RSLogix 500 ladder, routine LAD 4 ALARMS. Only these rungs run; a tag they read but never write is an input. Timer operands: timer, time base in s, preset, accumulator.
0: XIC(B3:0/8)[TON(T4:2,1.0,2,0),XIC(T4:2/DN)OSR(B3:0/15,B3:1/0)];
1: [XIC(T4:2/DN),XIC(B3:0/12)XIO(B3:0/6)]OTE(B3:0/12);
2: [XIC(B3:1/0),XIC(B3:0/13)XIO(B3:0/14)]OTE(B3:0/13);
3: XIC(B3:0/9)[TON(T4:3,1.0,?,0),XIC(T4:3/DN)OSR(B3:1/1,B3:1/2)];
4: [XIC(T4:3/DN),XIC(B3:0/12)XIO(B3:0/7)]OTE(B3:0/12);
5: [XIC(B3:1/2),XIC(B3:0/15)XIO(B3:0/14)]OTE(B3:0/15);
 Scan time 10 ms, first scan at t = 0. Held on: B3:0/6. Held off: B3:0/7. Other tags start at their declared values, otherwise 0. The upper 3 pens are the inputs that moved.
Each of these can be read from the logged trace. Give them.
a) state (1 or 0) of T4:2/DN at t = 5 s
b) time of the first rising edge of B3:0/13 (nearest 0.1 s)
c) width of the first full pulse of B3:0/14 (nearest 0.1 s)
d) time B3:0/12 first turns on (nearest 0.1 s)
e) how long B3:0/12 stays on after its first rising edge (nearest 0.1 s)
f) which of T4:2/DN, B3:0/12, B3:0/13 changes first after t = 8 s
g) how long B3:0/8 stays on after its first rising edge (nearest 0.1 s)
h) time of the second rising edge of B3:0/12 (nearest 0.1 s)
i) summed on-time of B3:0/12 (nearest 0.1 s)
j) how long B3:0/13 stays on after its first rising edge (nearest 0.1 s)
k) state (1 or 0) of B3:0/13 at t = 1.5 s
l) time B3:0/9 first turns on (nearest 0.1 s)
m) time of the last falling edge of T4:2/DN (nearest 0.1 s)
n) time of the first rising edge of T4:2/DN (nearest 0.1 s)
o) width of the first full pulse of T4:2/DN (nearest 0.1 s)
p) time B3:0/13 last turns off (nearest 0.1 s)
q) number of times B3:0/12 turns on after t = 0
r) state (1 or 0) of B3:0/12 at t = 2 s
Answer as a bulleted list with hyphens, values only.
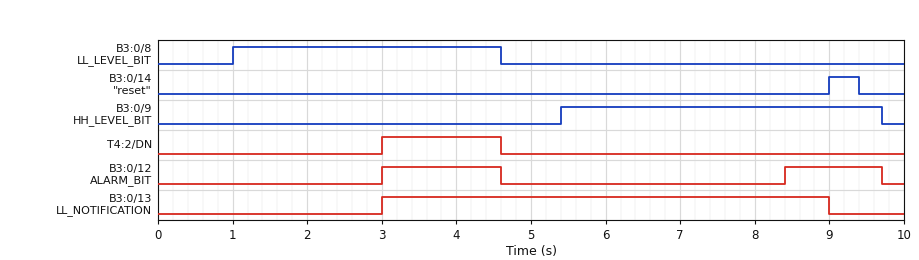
- 0
- 3.0 s
- 0.4 s
- 3.0 s
- 1.6 s
- B3:0/12
- 3.6 s
- 8.4 s
- 2.9 s
- 6.0 s
- 0
- 5.4 s
- 4.6 s
- 3.0 s
- 1.6 s
- 9.0 s
- 2
- 0
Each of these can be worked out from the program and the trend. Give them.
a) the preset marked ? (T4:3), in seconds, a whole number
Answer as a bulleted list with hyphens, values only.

- 3 s
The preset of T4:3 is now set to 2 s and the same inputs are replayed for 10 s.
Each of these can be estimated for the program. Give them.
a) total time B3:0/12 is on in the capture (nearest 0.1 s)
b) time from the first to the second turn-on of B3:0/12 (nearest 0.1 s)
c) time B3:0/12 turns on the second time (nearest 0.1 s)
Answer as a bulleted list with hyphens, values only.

- 3.9 s
- 4.4 s
- 7.4 s
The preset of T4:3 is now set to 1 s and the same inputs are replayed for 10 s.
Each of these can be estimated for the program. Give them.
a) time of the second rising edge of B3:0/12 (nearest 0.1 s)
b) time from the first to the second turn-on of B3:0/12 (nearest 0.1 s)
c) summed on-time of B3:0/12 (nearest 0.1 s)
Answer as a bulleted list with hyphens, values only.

- 6.4 s
- 3.4 s
- 4.9 s
